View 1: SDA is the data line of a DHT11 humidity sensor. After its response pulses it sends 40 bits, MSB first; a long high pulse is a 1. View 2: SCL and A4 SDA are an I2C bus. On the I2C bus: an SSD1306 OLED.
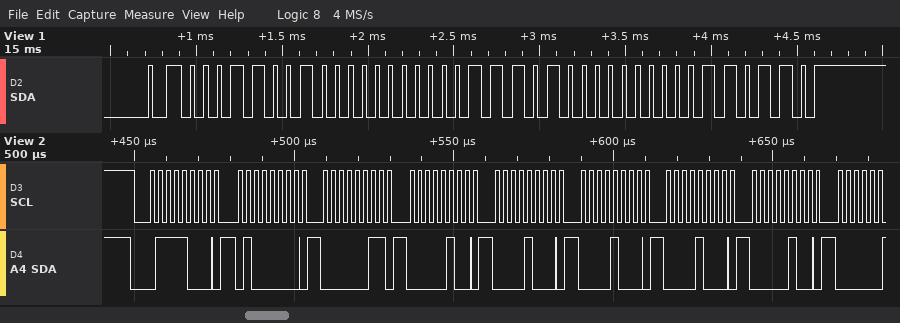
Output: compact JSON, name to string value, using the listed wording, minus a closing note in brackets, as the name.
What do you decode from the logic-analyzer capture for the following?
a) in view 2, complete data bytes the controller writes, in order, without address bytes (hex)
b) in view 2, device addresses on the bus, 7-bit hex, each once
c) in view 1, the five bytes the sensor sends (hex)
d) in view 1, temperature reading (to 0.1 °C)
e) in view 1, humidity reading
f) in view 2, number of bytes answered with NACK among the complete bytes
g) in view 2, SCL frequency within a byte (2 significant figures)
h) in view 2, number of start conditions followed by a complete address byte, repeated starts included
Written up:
{"in view 2, complete data bytes the controller writes, in order, without address bytes": "40 03 04 08 08 08 04", "in view 2, device addresses on the bus, 7-bit hex, each once": "0x3C", "in view 1, the five bytes the sensor sends": "19 00 1D 00 36", "in view 1, temperature reading": "29.0 °C", "in view 1, humidity reading": "25 %", "in view 2, number of bytes answered with NACK among the complete bytes": "0", "in view 2, SCL frequency within a byte": "400 kHz", "in view 2, number of start conditions followed by a complete address byte, repeated starts included": "1"}
